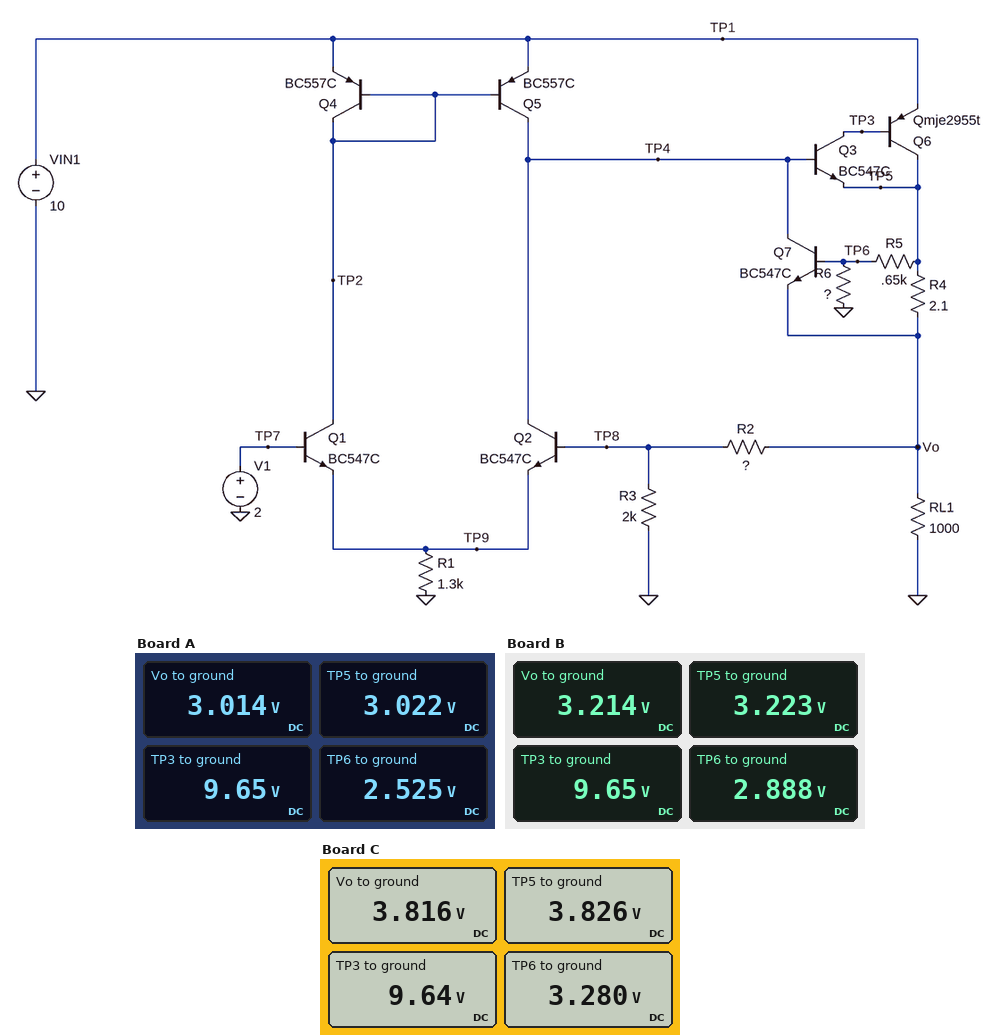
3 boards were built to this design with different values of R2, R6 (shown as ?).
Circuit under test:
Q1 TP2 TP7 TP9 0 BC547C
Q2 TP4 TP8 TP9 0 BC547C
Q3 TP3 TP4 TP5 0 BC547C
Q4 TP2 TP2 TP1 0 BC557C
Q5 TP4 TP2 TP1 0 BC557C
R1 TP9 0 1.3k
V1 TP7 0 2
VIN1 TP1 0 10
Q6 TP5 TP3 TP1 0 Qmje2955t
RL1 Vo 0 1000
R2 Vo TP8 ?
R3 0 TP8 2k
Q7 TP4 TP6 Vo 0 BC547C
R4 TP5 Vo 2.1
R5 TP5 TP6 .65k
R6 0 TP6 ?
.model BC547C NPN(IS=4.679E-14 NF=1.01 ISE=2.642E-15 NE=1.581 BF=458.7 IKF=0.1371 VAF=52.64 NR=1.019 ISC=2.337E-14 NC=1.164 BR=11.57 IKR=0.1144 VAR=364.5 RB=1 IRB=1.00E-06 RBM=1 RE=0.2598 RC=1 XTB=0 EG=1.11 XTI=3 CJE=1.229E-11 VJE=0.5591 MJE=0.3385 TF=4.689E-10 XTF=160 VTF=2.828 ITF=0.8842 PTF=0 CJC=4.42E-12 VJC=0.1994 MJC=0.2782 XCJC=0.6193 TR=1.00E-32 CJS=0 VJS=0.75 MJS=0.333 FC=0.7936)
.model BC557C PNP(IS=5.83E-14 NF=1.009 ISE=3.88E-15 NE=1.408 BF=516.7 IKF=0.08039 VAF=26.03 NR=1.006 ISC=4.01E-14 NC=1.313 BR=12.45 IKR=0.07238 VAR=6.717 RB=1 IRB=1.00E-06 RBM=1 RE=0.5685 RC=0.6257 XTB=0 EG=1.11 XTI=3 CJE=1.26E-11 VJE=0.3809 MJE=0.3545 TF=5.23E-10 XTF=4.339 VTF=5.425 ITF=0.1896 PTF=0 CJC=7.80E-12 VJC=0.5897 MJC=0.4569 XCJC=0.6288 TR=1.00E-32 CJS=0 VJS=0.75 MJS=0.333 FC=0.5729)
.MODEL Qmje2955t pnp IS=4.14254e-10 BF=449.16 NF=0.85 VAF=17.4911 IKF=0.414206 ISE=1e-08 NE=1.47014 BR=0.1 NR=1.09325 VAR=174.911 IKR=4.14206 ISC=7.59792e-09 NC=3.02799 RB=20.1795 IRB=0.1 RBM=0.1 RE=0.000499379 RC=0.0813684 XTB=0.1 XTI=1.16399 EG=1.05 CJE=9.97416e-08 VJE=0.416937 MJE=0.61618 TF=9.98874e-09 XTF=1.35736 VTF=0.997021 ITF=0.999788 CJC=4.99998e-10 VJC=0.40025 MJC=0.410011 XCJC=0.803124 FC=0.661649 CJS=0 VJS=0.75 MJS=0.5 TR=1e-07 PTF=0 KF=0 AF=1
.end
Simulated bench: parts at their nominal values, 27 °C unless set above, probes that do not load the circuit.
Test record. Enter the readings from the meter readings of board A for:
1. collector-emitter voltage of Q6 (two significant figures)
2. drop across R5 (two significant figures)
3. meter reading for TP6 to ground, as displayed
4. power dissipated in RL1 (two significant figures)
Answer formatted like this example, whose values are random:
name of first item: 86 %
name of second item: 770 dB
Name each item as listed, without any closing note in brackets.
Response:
collector-emitter voltage of Q6: -7.0 V
drop across R5: 500 mV
meter reading for TP6 to ground, as displayed: 2.525 V
power dissipated in RL1: 9.1 mW
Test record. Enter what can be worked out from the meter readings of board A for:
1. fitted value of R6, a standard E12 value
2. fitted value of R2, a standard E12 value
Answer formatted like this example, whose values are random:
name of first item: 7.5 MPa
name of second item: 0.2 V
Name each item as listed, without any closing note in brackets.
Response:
fitted value of R6, a standard E12 value: 3.3 kΩ
fitted value of R2, a standard E12 value: 1 kΩ
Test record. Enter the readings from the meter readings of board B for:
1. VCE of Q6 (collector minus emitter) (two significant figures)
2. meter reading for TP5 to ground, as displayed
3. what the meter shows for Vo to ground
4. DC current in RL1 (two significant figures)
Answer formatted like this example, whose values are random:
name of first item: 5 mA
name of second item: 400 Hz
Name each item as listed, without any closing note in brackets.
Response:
VCE of Q6 (collector minus emitter): -6.8 V
meter reading for TP5 to ground, as displayed: 3.223 V
what the meter shows for Vo to ground: 3.214 V
DC current in RL1: 3.2 mA
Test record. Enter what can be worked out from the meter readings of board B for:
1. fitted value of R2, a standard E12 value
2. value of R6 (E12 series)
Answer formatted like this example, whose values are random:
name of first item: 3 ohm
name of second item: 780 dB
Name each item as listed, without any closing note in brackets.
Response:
fitted value of R2, a standard E12 value: 1.2 kΩ
value of R6: 5.6 kΩ
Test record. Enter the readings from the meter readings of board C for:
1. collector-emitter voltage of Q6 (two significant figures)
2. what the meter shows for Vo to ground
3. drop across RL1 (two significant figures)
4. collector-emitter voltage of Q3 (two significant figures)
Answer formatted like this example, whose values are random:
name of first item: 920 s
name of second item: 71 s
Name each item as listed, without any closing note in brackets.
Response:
collector-emitter voltage of Q6: -6.2 V
what the meter shows for Vo to ground: 3.816 V
drop across RL1: 3.8 V
collector-emitter voltage of Q3: 5.8 V
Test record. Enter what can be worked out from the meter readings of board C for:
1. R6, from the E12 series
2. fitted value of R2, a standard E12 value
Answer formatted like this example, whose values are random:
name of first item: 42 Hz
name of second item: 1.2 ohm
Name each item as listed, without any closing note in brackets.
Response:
R6, from the E12 series: 3.9 kΩ
fitted value of R2, a standard E12 value: 1.8 kΩ
